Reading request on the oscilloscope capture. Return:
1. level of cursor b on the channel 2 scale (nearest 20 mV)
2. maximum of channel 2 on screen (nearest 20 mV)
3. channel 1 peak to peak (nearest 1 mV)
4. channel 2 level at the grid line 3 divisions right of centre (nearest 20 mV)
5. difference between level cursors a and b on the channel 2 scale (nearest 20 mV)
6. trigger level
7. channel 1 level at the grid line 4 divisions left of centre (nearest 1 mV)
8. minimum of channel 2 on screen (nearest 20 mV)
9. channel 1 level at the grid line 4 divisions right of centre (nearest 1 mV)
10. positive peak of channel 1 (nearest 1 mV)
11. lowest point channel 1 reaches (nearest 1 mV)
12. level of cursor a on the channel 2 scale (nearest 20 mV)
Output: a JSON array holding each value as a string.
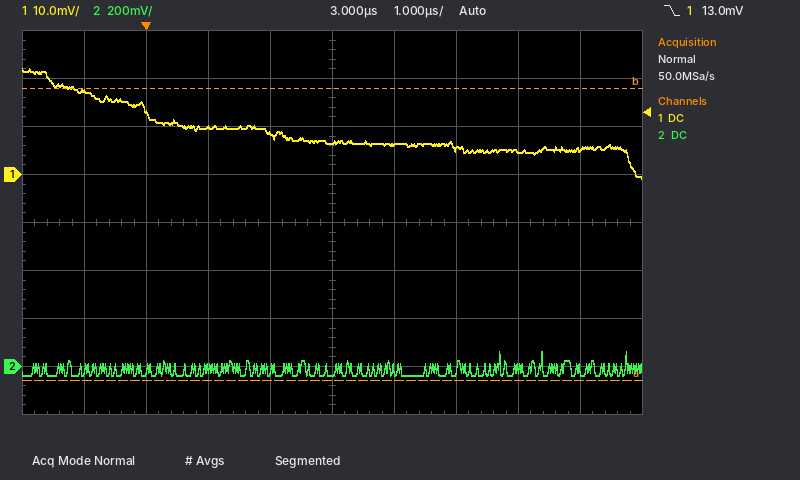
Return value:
["1.16 V", "60 mV", "23 mV", "0 mV", "1.22 V", "13.0 mV", "17 mV", "-40 mV", "5 mV", "22 mV", "-1 mV", "-60 mV"]
